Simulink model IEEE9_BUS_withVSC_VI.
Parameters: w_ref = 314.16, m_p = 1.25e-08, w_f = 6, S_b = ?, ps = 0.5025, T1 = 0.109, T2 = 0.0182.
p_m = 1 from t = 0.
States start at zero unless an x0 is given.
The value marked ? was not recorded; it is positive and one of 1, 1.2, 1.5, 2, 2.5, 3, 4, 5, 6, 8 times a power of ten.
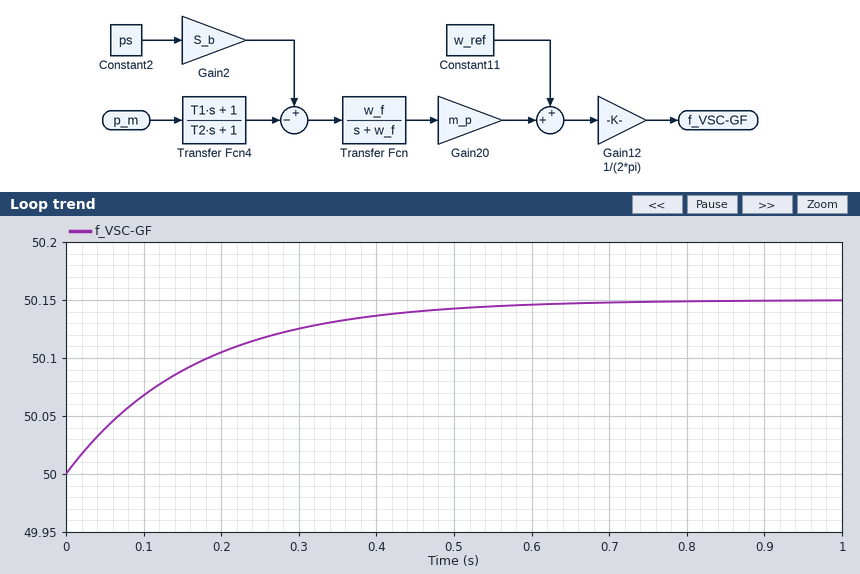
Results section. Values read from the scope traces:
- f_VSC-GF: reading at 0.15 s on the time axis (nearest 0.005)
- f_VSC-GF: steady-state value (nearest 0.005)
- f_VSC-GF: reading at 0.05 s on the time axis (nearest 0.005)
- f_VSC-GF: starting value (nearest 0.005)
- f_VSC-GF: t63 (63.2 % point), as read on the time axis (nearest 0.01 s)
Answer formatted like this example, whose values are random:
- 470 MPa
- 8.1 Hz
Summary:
- 50.090
- 50.150
- 50.040
- 50.000
- 0.17 s
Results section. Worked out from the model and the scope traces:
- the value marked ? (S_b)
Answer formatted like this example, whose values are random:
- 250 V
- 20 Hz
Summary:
- 1.5e+08
